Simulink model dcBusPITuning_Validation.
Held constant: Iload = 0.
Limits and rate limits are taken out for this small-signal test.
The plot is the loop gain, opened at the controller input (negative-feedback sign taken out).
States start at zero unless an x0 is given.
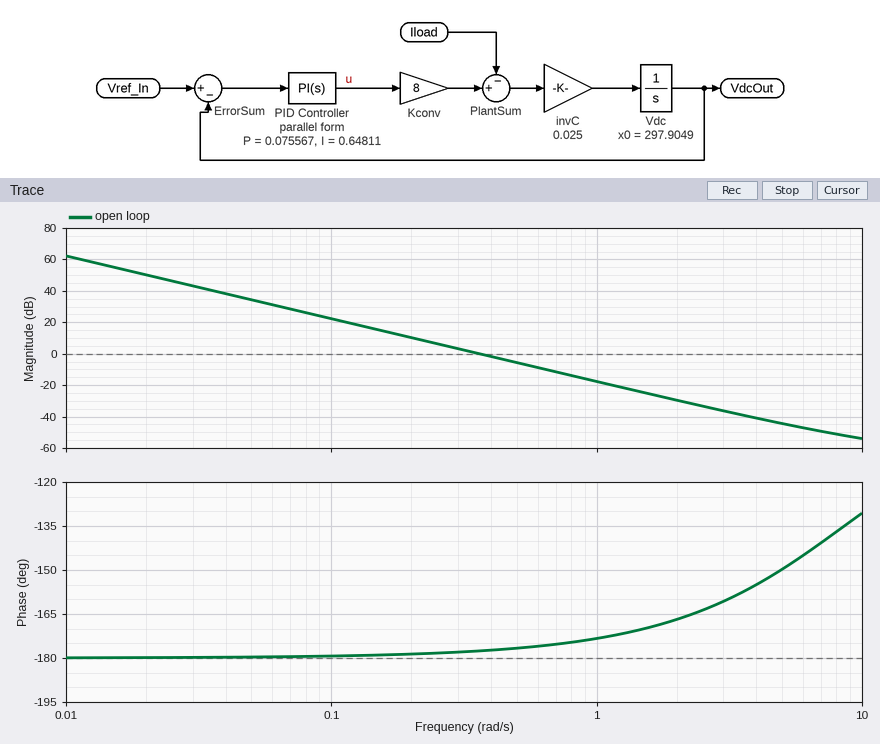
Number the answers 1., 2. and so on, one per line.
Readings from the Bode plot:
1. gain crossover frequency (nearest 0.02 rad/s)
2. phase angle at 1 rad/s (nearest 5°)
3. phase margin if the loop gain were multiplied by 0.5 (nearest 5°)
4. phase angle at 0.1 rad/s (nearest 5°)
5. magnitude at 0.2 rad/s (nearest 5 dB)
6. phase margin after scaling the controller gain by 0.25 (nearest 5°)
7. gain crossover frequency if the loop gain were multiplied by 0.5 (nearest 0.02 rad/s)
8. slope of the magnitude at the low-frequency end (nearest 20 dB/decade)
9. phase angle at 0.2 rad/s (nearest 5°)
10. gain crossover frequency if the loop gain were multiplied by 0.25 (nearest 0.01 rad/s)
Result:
1. 0.36 rad/s
2. -175°
3. 0°
4. -180°
5. 10 dB
6. 0°
7. 0.26 rad/s
8. -40 dB/decade
9. -180°
10. 0.18 rad/s
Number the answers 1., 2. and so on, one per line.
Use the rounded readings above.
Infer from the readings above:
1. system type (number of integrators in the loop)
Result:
1. 2
